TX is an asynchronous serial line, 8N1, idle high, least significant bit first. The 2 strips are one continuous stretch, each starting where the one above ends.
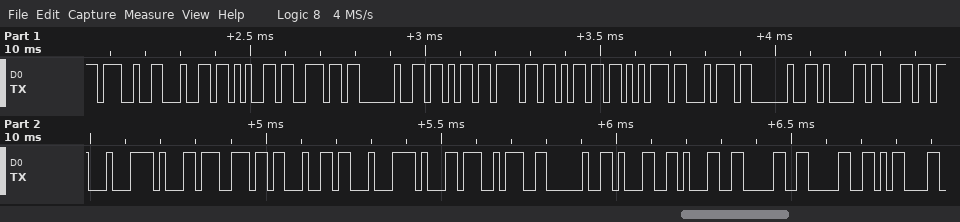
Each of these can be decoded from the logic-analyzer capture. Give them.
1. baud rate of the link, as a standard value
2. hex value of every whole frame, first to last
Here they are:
57600 baud
0x27 0x64 0x65 0x6E 0x20 0x6B 0x6F 0x6D 0x75 0x74 0x20 0x61 0x6C 0xC4 0xB1 0x6E 0x64 0xC4 0xB1 0x3A 0x20 0x31 0x31 0x30 0x30 0x0D
